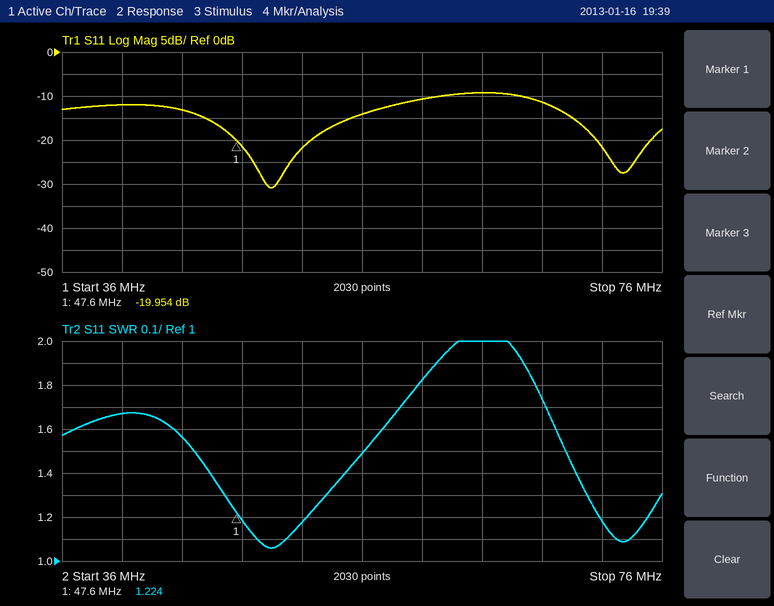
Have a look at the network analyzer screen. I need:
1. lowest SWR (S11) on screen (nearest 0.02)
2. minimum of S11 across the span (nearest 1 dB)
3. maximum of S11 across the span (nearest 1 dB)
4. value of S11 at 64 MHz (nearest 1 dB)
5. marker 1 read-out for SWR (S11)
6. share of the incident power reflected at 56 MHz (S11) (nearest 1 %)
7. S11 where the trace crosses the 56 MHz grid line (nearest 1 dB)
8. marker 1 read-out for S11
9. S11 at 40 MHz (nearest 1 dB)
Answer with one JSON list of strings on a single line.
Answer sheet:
["1.06", "-31 dB", "-9 dB", "-9 dB", "1.224", "4 %", "-14 dB", "-19.954 dB", "-12 dB"]
